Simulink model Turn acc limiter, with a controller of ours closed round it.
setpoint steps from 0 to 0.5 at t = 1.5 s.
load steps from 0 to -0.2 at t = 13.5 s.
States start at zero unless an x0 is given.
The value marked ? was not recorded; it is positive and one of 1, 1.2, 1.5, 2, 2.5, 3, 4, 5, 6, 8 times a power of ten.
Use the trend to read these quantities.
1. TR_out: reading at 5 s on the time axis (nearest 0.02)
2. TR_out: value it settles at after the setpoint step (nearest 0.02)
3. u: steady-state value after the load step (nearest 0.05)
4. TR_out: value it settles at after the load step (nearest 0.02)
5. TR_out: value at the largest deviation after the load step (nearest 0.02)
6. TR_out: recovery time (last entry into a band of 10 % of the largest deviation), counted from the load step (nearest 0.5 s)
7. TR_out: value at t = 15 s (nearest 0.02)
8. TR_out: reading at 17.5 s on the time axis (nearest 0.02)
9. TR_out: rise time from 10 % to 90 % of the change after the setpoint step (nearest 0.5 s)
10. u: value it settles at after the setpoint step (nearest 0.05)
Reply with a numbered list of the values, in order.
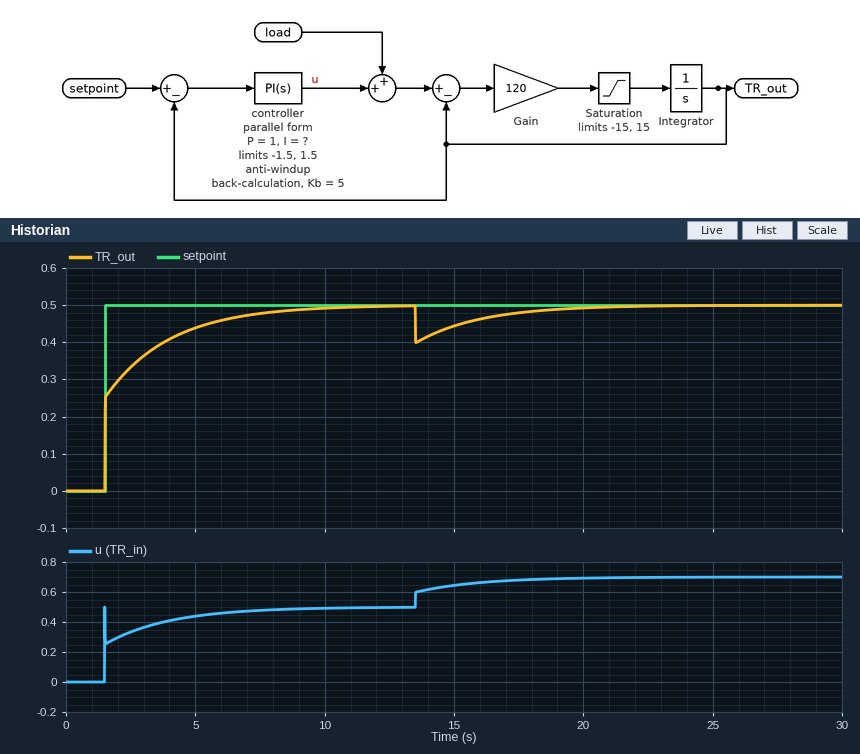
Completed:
1. 0.44
2. 0.50
3. 0.70
4. 0.50
5. 0.40
6. 6.0 s
7. 0.44
8. 0.48
9. 4.0 s
10. 0.50
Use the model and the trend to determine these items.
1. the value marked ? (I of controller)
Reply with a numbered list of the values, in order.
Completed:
1. 0.8
